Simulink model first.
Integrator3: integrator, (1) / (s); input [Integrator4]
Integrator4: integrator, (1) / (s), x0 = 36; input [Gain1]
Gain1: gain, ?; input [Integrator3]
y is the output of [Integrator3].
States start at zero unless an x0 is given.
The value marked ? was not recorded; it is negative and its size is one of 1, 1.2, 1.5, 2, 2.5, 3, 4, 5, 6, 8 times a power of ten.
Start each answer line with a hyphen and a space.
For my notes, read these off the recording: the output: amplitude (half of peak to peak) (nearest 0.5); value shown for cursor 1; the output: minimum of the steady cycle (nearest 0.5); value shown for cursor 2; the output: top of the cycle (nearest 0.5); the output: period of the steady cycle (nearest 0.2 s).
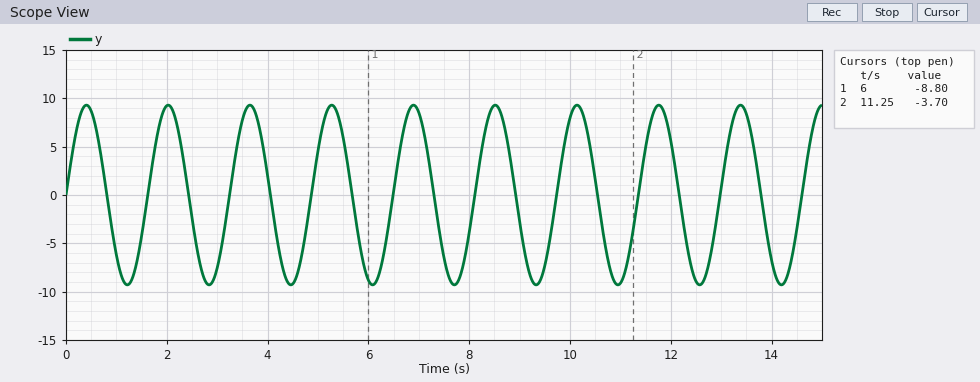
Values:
- 9.5
- -8.80
- -9.5
- -3.70
- 9.5
- 1.6 s
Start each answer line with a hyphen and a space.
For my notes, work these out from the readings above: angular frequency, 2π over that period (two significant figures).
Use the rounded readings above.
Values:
- 3.9 rad/s
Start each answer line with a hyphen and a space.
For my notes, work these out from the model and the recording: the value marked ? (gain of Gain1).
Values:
- -15
